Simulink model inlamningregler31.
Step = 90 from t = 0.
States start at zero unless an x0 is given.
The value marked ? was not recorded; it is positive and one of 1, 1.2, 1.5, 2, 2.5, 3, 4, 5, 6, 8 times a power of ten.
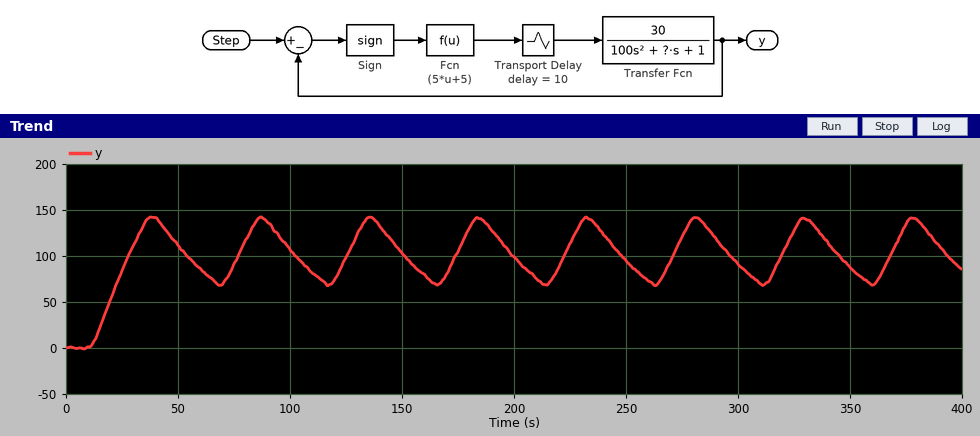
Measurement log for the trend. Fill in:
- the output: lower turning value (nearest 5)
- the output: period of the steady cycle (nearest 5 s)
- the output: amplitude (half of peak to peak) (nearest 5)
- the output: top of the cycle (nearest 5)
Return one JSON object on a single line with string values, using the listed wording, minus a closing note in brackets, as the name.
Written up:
{"the output: lower turning value": "70", "the output: period of the steady cycle": "50 s", "the output: amplitude (half of peak to peak)": "35", "the output: top of the cycle": "140"}
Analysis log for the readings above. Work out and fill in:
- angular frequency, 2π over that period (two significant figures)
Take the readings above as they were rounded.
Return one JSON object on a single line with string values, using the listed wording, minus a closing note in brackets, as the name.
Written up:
{"angular frequency, 2π over that period": "0.13 rad/s"}
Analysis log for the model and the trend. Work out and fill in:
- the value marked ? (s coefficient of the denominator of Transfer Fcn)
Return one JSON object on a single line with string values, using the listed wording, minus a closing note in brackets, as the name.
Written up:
{"the value marked ?": "40"}
